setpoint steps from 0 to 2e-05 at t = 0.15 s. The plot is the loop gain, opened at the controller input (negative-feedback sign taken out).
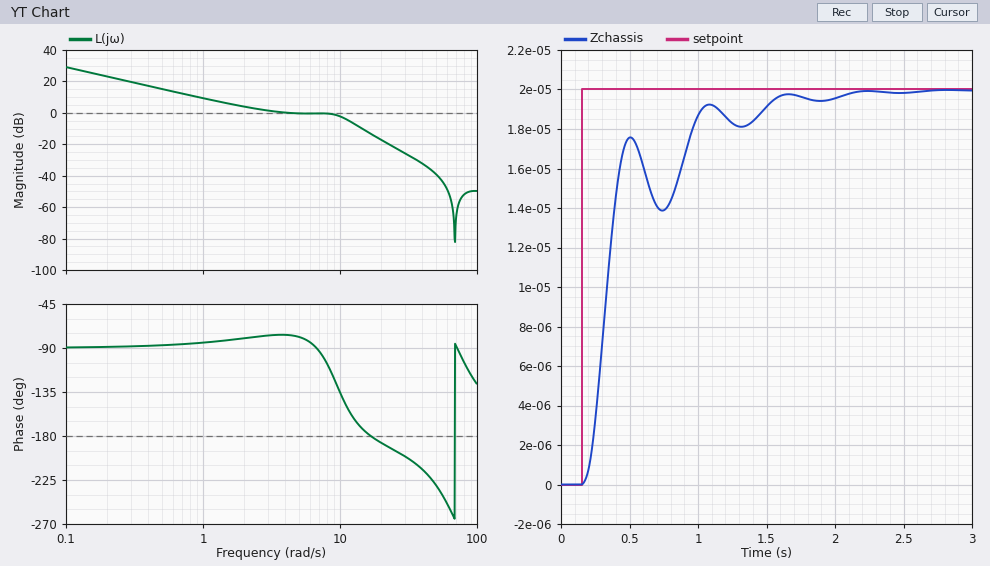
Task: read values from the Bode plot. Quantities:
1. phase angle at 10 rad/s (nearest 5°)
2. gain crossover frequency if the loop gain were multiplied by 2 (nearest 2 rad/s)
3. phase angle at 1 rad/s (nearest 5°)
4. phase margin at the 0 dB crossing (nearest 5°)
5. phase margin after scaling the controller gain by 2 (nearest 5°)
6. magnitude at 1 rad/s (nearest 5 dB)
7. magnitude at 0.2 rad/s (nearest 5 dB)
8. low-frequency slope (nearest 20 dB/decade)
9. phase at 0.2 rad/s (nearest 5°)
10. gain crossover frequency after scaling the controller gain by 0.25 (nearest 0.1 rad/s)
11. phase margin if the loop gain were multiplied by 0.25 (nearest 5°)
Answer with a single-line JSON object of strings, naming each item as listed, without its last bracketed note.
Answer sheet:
{"phase angle at 10 rad/s": "-135°", "gain crossover frequency if the loop gain were multiplied by 2": "12 rad/s", "phase angle at 1 rad/s": "-85°", "phase margin at the 0 dB crossing": "105°", "phase margin after scaling the controller gain by 2": "20°", "magnitude at 1 rad/s": "10 dB", "magnitude at 0.2 rad/s": "25 dB", "low-frequency slope": "-20 dB/decade", "phase at 0.2 rad/s": "-90°", "gain crossover frequency after scaling the controller gain by 0.25": "0.7 rad/s", "phase margin if the loop gain were multiplied by 0.25": "95°"}
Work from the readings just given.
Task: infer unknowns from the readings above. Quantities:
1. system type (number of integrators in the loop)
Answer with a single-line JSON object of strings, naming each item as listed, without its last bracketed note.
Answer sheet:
{"system type": "1"}
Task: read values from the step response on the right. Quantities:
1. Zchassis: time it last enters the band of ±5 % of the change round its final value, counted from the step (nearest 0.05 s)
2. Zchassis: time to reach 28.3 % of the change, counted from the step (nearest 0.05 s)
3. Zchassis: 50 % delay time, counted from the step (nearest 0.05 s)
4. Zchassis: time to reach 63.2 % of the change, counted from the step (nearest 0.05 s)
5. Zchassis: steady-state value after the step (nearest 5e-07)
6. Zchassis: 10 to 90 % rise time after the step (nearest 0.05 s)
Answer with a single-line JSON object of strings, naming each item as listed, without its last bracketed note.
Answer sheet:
{"Zchassis: time it last enters the band of ±5 % of the change round its final value, counted from the step": "1.35 s", "Zchassis: time to reach 28.3 % of the change, counted from the step": "0.15 s", "Zchassis: 50 % delay time, counted from the step": "0.20 s", "Zchassis: time to reach 63.2 % of the change, counted from the step": "0.20 s", "Zchassis: steady-state value after the step": "0.0000200", "Zchassis: 10 to 90 % rise time after the step": "0.75 s"}
